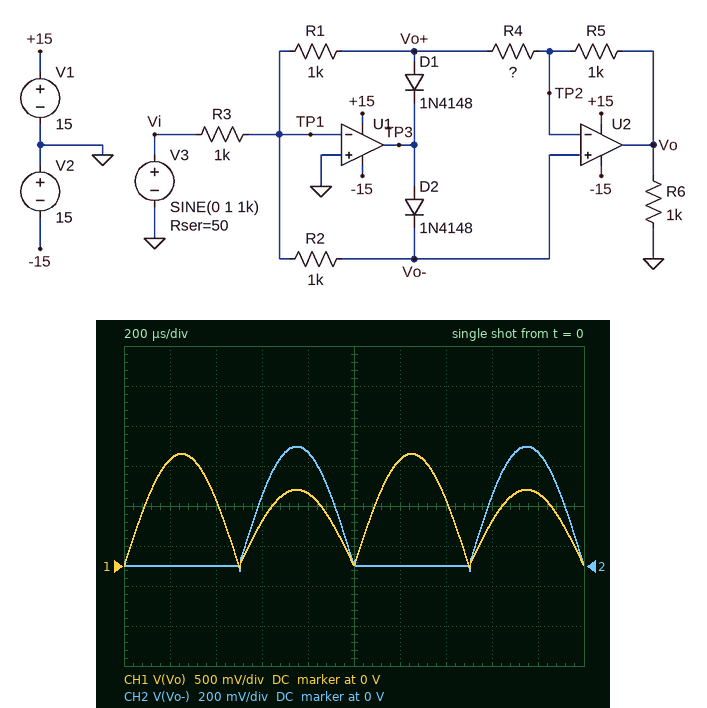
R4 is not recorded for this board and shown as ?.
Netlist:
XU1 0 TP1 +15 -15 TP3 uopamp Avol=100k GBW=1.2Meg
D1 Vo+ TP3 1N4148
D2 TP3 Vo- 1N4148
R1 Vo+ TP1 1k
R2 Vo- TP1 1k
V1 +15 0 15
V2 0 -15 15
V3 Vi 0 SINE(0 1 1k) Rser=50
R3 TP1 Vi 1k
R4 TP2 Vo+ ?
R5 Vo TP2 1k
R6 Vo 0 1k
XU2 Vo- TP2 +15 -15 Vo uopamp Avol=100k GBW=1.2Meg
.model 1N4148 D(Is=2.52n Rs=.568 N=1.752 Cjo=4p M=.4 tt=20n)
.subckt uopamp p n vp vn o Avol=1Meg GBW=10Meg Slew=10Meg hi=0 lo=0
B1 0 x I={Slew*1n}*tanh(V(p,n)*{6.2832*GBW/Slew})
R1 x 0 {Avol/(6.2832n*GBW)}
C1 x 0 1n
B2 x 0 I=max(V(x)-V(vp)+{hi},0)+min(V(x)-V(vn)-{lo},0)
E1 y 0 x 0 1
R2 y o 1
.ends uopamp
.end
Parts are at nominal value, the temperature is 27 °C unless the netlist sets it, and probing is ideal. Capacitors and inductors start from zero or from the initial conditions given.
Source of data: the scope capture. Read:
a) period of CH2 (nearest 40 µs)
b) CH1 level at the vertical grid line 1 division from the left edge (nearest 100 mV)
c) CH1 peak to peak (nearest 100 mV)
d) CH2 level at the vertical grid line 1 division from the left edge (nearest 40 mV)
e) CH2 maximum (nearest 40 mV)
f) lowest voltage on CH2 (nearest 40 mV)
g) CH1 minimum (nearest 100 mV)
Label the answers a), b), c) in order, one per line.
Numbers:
a) 1.00 ms
b) 1.3 V
c) 1.4 V
d) 0 V
e) 600 mV
f) -40 mV
g) 0 V
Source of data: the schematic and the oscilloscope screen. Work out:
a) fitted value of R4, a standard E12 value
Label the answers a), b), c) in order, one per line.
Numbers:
a) 680 Ω
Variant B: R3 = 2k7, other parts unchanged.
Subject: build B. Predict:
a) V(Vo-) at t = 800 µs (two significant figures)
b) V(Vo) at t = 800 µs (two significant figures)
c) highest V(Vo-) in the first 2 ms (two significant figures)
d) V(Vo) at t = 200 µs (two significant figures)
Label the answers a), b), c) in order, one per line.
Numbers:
a) 220 mV
b) 350 mV
c) 230 mV
d) 510 mV
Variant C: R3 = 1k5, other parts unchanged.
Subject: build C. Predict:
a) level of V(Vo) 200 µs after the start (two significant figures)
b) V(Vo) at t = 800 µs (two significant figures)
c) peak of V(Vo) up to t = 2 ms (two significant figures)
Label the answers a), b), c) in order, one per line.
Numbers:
a) 900 mV
b) 610 mV
c) 950 mV
